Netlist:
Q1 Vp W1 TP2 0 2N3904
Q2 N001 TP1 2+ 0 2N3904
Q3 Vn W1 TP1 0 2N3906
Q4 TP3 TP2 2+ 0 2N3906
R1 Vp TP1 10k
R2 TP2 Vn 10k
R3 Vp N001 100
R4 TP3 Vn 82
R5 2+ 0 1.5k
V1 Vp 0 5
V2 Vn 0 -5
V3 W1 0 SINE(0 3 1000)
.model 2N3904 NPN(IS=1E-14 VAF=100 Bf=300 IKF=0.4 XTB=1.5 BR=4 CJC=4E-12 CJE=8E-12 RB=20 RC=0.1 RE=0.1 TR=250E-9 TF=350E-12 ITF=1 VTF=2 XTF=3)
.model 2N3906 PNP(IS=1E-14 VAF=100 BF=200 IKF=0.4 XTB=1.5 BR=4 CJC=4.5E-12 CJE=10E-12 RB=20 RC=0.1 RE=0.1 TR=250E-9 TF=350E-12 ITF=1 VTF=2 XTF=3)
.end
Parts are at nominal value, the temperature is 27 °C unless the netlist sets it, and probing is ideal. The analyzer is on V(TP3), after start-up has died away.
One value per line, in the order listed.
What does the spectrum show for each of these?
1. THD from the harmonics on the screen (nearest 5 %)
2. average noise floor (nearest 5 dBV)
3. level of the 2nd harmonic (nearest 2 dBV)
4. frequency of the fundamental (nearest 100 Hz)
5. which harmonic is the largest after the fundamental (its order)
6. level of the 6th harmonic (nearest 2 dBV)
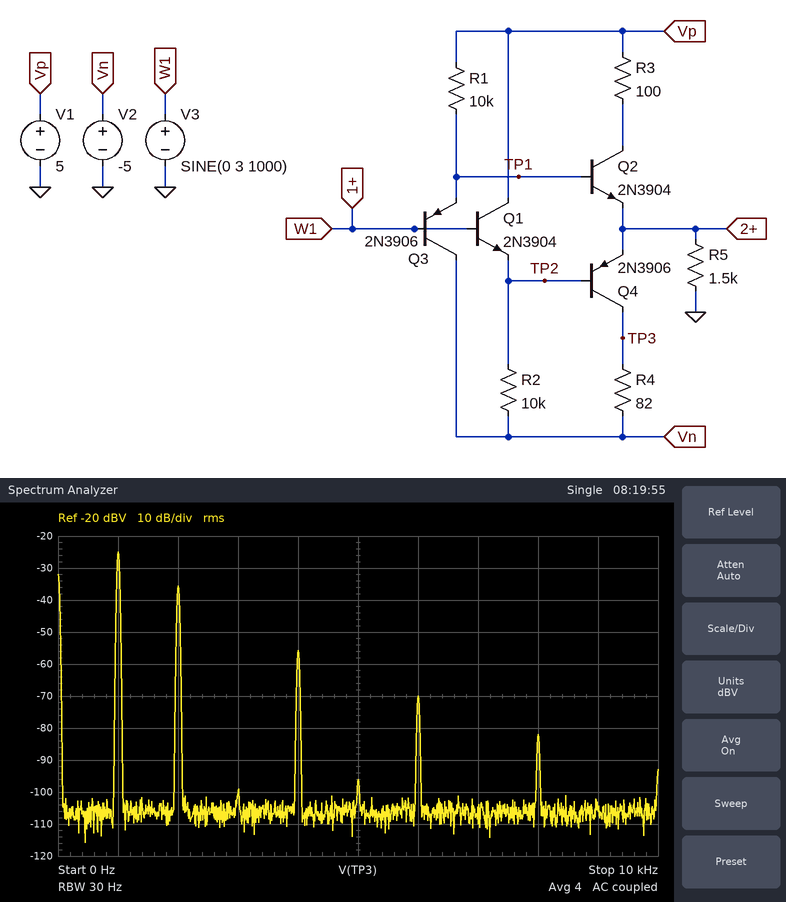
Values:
30 %
-105 dBV
-36 dBV
1.0 kHz
2
-70 dBV
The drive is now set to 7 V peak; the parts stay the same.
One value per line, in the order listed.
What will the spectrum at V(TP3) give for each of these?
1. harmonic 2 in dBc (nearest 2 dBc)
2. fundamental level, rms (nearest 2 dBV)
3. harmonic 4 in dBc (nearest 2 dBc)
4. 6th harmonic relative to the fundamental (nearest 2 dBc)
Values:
-12 dBc
-20 dBV
-16 dBc
-26 dBc
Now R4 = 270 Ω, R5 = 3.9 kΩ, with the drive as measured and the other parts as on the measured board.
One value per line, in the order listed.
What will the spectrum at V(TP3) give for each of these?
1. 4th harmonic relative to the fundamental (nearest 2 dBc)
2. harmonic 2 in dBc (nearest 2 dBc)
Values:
-58 dBc
-22 dBc
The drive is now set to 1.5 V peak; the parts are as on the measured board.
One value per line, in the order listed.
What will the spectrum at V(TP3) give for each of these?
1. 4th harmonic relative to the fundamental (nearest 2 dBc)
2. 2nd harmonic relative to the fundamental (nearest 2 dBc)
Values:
-40 dBc
-14 dBc
